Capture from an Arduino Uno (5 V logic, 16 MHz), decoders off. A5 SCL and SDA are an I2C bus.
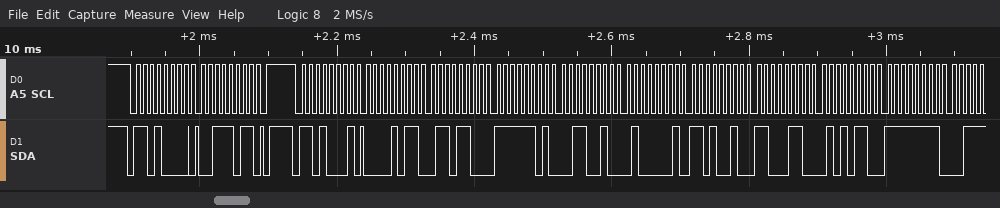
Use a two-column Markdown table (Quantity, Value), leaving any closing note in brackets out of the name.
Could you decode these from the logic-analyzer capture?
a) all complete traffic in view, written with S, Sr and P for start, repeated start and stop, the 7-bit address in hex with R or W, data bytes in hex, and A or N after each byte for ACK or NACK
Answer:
| Quantity | Value |
|---|---|
| all complete traffic in view, written with S, Sr and P for start, repeated start and stop, the 7-bit address in hex with R or W, data bytes in hex, and A or N after each byte for ACK or NACK | S 68W A 3B A P S 68R A 0B A 6C A FD A 32 A 41 A D2 A C6 A 56 A FF A |
